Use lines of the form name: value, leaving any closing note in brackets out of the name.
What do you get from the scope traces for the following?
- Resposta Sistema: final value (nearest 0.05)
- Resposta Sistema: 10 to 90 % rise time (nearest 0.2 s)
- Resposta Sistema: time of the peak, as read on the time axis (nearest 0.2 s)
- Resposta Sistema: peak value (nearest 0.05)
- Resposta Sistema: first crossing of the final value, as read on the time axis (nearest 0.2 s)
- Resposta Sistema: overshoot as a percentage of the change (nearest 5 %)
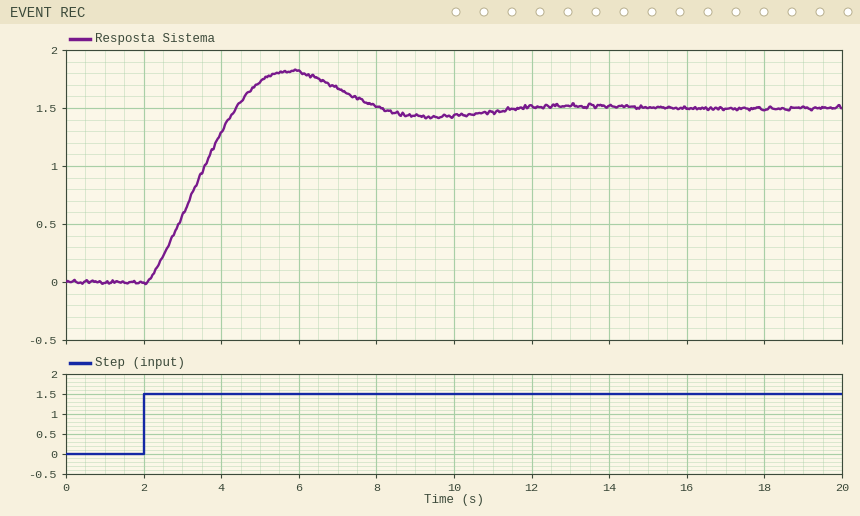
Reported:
Resposta Sistema: final value: 1.50
Resposta Sistema: 10 to 90 % rise time: 1.8 s
Resposta Sistema: time of the peak, as read on the time axis: 5.8 s
Resposta Sistema: peak value: 1.80
Resposta Sistema: first crossing of the final value, as read on the time axis: 4.4 s
Resposta Sistema: overshoot as a percentage of the change: 20 %
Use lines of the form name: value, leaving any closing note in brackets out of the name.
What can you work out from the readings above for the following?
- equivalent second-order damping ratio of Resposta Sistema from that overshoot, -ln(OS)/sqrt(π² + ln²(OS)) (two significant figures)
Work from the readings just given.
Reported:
equivalent second-order damping ratio of Resposta Sistema from that overshoot, -ln(OS)/sqrt(π² + ln²(OS)): 0.46
